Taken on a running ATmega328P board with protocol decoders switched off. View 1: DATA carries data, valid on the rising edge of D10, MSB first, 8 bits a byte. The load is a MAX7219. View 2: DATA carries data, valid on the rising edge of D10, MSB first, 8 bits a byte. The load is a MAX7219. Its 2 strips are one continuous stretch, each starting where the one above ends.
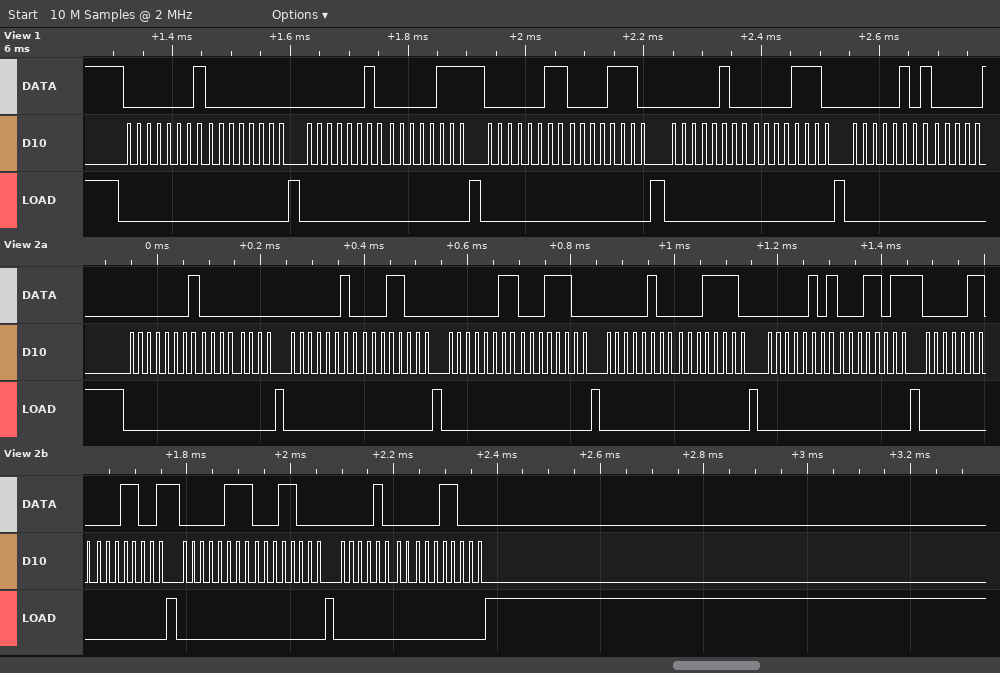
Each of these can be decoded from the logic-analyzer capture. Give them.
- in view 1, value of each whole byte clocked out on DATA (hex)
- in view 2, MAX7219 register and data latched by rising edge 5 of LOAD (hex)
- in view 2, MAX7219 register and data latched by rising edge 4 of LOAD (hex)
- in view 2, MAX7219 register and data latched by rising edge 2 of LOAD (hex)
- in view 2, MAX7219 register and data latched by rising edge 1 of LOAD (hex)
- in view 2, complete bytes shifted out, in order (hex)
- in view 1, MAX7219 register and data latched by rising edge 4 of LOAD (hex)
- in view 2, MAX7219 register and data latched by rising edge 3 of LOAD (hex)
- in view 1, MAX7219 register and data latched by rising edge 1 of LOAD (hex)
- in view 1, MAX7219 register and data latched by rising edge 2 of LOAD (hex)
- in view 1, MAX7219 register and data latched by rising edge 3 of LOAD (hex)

0x01 0x00 0x02 0x07 0x03 0x0E 0x04 0x0E 0x05
register 0x5, data 0x1B
register 0x4, data 0x1E
register 0x2, data 0x18
register 0x1, data 0x00
01 00 02 18 03 1C 04 1E 05 1B 06 19 07 18 08 18
register 0x4, data 0x0E
register 0x3, data 0x1C
register 0x1, data 0x00
register 0x2, data 0x07
register 0x3, data 0x0E
